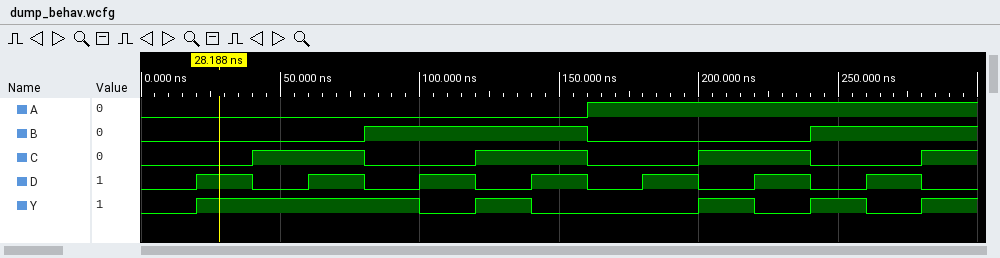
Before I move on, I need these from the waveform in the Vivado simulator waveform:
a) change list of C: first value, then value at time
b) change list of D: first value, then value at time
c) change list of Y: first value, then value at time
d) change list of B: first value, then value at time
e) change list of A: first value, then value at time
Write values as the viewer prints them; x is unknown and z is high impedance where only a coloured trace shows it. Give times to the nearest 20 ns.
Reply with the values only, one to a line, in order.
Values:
0, 1 at 40 ns, 0 at 80 ns, 1 at 120 ns, 0 at 160 ns, 1 at 200 ns, 0 at 240 ns, 1 at 280 ns
0, 1 at 20 ns, 0 at 40 ns, 1 at 60 ns, 0 at 80 ns, 1 at 100 ns, 0 at 120 ns, 1 at 140 ns, 0 at 160 ns, 1 at 180 ns, 0 at 200 ns, 1 at 220 ns, 0 at 240 ns, 1 at 260 ns, 0 at 280 ns
0, 1 at 20 ns, 0 at 100 ns, 1 at 120 ns, 0 at 140 ns, 1 at 200 ns, 0 at 220 ns, 1 at 240 ns, 0 at 260 ns, 1 at 280 ns
0, 1 at 80 ns, 0 at 160 ns, 1 at 240 ns
0, 1 at 160 ns
